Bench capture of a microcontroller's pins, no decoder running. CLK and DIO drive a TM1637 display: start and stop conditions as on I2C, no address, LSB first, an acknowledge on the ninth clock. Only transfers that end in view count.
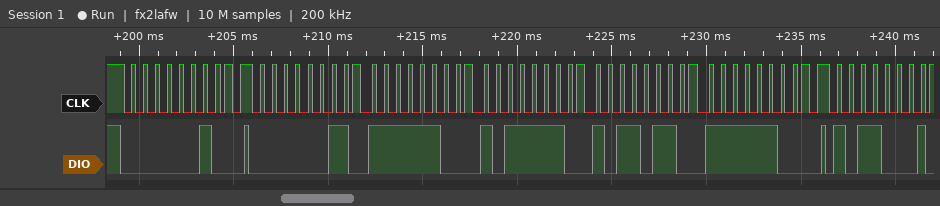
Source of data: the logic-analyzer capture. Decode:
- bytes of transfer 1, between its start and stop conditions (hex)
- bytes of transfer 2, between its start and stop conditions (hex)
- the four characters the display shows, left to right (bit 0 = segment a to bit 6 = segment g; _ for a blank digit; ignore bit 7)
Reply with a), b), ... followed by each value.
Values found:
a) 40
b) C0 3F 7D 6D 3F
c) 0650
